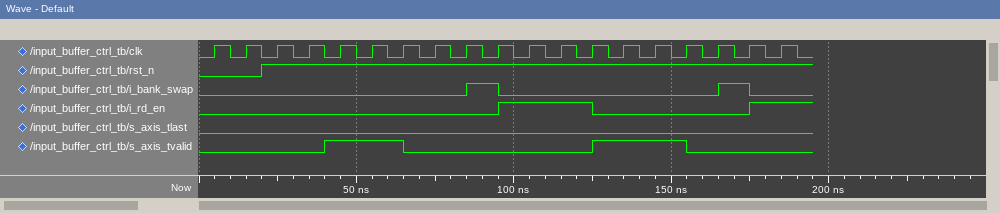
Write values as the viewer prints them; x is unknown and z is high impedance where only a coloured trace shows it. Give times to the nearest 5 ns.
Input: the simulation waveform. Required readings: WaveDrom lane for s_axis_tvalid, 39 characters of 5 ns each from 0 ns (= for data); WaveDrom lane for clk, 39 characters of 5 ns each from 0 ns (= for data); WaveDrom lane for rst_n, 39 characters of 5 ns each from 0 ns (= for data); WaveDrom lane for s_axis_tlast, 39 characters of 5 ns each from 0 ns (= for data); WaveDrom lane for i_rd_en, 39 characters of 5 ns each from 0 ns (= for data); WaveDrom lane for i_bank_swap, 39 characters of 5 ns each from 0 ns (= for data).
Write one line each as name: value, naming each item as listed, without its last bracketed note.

WaveDrom lane for s_axis_tvalid, 39 characters of 5 ns each from 0 ns: {name: 's_axis_tvalid', wave: '0.......1....0...........1.....0.......'}
WaveDrom lane for clk, 39 characters of 5 ns each from 0 ns: {name: 'clk', wave: '010101010101010101010101010101010101010'}
WaveDrom lane for rst_n, 39 characters of 5 ns each from 0 ns: {name: 'rst_n', wave: '0...1..................................'}
WaveDrom lane for s_axis_tlast, 39 characters of 5 ns each from 0 ns: {name: 's_axis_tlast', wave: '0......................................'}
WaveDrom lane for i_rd_en, 39 characters of 5 ns each from 0 ns: {name: 'i_rd_en', wave: '0..................1.....0.........1...'}
WaveDrom lane for i_bank_swap, 39 characters of 5 ns each from 0 ns: {name: 'i_bank_swap', wave: '0................1.0.............1.0...'}
